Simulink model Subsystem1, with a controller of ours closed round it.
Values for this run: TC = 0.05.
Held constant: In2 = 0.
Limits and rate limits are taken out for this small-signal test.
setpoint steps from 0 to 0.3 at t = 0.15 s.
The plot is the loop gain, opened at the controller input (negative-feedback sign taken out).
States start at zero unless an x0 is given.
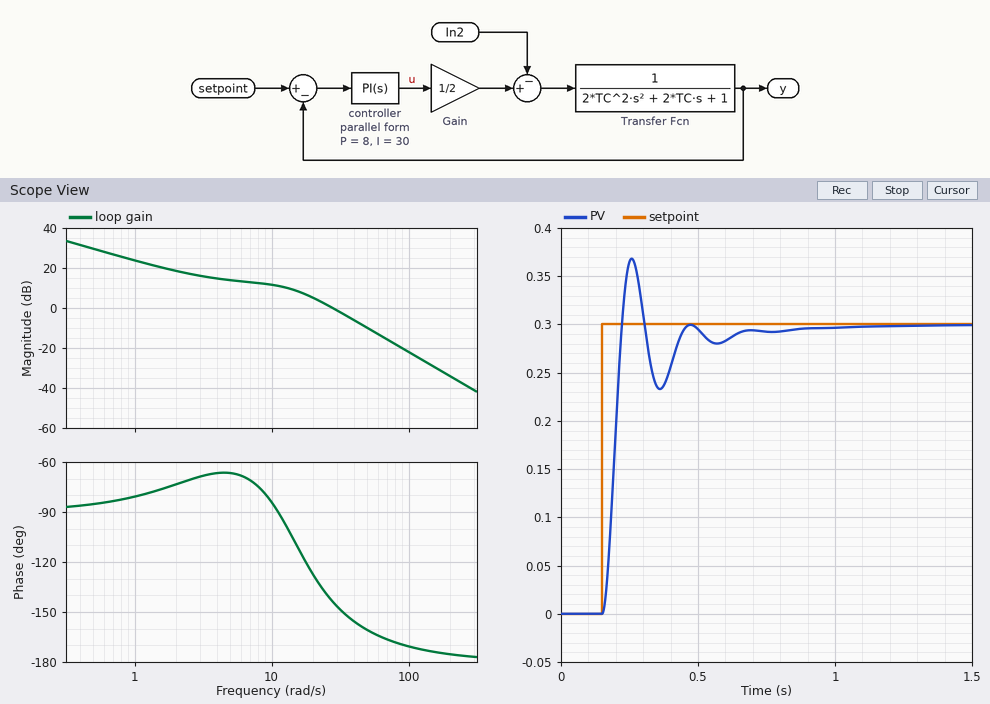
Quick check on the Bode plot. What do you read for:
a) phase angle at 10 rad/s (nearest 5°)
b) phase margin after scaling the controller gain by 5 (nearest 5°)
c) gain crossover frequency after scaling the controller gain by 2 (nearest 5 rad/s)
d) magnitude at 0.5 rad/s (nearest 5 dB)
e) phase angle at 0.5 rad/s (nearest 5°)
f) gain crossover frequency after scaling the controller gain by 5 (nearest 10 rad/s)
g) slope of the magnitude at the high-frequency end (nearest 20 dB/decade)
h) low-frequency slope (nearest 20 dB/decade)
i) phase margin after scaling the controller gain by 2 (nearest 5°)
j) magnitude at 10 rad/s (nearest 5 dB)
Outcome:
-85°
15°
40 rad/s
30 dB
-85°
60 rad/s
-40 dB/decade
-20 dB/decade
25°
10 dB
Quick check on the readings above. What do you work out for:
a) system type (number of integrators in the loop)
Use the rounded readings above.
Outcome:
1
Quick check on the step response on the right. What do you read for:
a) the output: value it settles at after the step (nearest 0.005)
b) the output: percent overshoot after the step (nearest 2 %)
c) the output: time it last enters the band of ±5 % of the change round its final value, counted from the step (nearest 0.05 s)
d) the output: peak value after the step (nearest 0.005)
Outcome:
0.300
22 %
0.45 s
0.370
